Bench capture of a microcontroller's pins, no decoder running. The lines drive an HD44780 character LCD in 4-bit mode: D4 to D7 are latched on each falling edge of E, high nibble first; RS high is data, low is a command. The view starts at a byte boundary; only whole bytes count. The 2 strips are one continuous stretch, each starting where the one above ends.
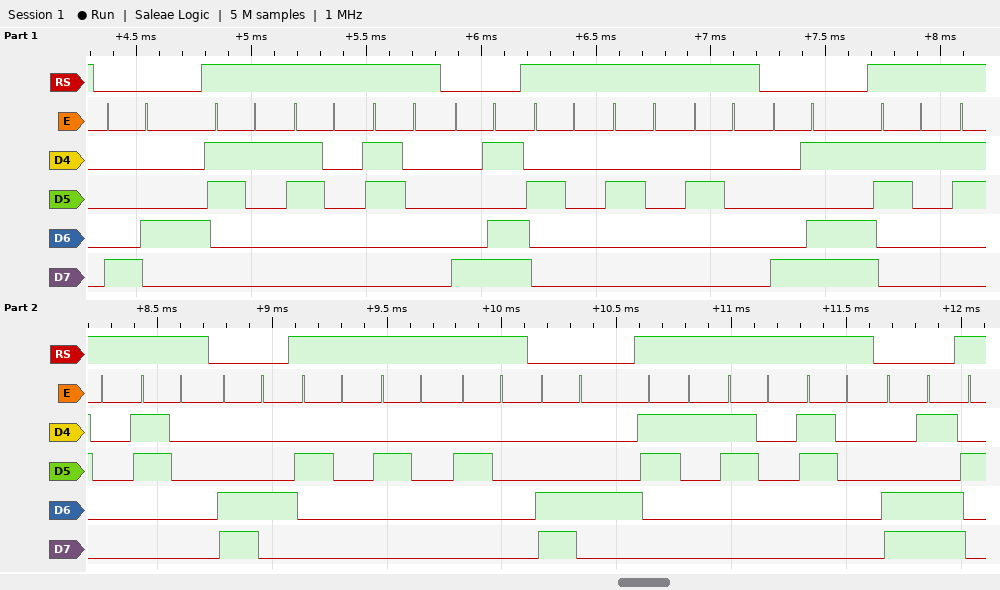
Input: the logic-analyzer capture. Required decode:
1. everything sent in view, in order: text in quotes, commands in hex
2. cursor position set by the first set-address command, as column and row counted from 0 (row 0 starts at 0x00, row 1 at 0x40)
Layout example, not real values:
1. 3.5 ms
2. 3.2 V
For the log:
1. 0x84 "100" 0x8D "   " 0x8D "100" 0xC4 "   " 0xC4 "100" 0xCD
2. column 4, row 0
